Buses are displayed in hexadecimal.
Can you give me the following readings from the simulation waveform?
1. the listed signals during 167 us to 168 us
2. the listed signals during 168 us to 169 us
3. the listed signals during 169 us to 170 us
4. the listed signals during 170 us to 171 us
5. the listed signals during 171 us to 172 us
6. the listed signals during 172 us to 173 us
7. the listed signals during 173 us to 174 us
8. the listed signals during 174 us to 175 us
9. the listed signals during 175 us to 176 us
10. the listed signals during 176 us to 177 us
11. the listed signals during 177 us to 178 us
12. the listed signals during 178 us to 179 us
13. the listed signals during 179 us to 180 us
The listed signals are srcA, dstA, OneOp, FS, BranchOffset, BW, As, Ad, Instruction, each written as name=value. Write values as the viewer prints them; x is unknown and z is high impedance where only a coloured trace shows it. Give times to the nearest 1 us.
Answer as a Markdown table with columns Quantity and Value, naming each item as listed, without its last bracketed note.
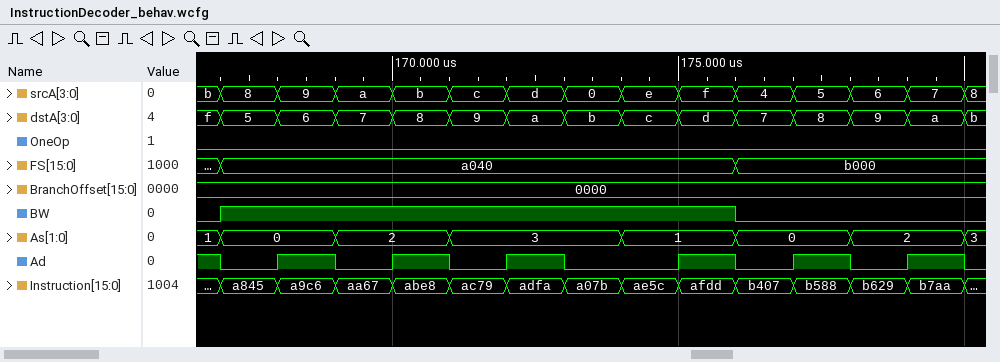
| Quantity | Value |
|---|---|
| the listed signals during 167 us to 168 us | srcA=8, dstA=5, OneOp=0, FS=a040, BranchOffset=0000, BW=1, As=0, Ad=0, Instruction=a845 |
| the listed signals during 168 us to 169 us | srcA=9, dstA=6, OneOp=0, FS=a040, BranchOffset=0000, BW=1, As=0, Ad=1, Instruction=a9c6 |
| the listed signals during 169 us to 170 us | srcA=a, dstA=7, OneOp=0, FS=a040, BranchOffset=0000, BW=1, As=2, Ad=0, Instruction=aa67 |
| the listed signals during 170 us to 171 us | srcA=b, dstA=8, OneOp=0, FS=a040, BranchOffset=0000, BW=1, As=2, Ad=1, Instruction=abe8 |
| the listed signals during 171 us to 172 us | srcA=c, dstA=9, OneOp=0, FS=a040, BranchOffset=0000, BW=1, As=3, Ad=0, Instruction=ac79 |
| the listed signals during 172 us to 173 us | srcA=d, dstA=a, OneOp=0, FS=a040, BranchOffset=0000, BW=1, As=3, Ad=1, Instruction=adfa |
| the listed signals during 173 us to 174 us | srcA=0, dstA=b, OneOp=0, FS=a040, BranchOffset=0000, BW=1, As=3, Ad=0, Instruction=a07b |
| the listed signals during 174 us to 175 us | srcA=e, dstA=c, OneOp=0, FS=a040, BranchOffset=0000, BW=1, As=1, Ad=0, Instruction=ae5c |
| the listed signals during 175 us to 176 us | srcA=f, dstA=d, OneOp=0, FS=a040, BranchOffset=0000, BW=1, As=1, Ad=1, Instruction=afdd |
| the listed signals during 176 us to 177 us | srcA=4, dstA=7, OneOp=0, FS=b000, BranchOffset=0000, BW=0, As=0, Ad=0, Instruction=b407 |
| the listed signals during 177 us to 178 us | srcA=5, dstA=8, OneOp=0, FS=b000, BranchOffset=0000, BW=0, As=0, Ad=1, Instruction=b588 |
| the listed signals during 178 us to 179 us | srcA=6, dstA=9, OneOp=0, FS=b000, BranchOffset=0000, BW=0, As=2, Ad=0, Instruction=b629 |
| the listed signals during 179 us to 180 us | srcA=7, dstA=a, OneOp=0, FS=b000, BranchOffset=0000, BW=0, As=2, Ad=1, Instruction=b7aa |
